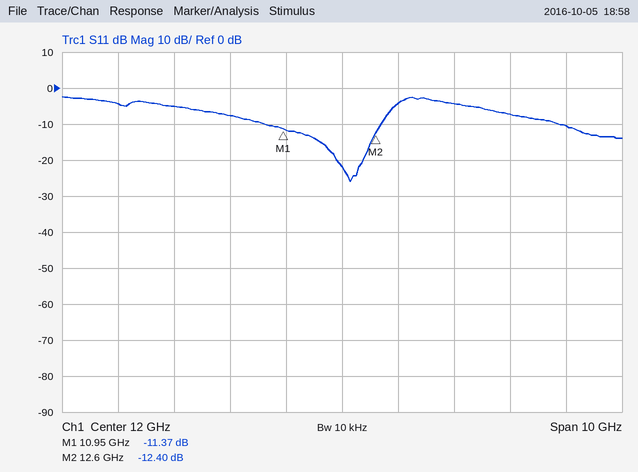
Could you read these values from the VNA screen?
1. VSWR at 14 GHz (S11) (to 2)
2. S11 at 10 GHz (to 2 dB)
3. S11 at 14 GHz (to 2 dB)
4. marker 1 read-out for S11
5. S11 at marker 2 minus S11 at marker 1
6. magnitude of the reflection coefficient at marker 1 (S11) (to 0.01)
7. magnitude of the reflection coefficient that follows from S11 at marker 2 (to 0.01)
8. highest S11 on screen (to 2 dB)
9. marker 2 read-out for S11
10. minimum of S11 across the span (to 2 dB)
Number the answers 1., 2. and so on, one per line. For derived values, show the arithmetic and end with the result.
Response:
1. |Γ| = 10^(-4/20) = 0.6310; VSWR = (1 + 0.6310)/(1 − 0.6310) ≈ 4
2. -8 dB
3. -4 dB
4. -11.37 dB
5. -12.4 − (-11.37) = -1.03 dB
6. 10^(-11.37/20) ≈ 0.27
7. 10^(-12.4/20) ≈ 0.24
8. -2 dB
9. -12.40 dB
10. -26 dB
